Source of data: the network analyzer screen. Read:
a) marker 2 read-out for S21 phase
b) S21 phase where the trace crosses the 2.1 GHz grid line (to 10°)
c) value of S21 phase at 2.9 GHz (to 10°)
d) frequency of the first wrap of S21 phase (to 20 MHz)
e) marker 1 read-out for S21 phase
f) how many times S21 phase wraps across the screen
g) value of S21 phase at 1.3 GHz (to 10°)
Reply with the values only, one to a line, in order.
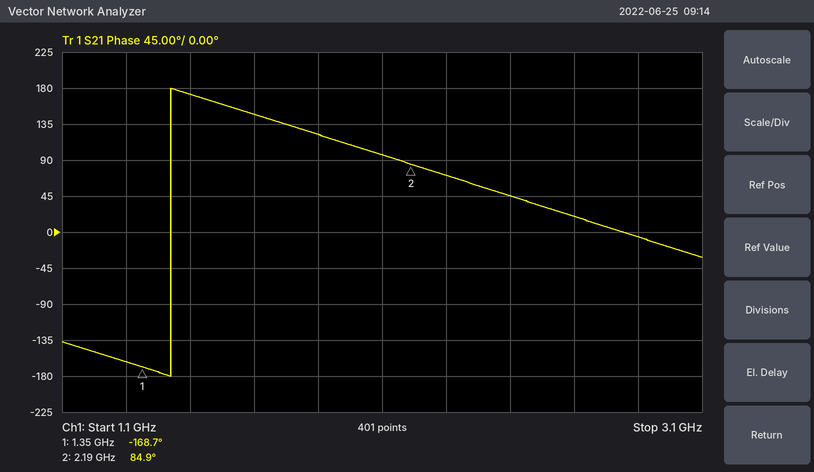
84.9°
100°
-10°
1.44 GHz
-168.7°
1
-160°
